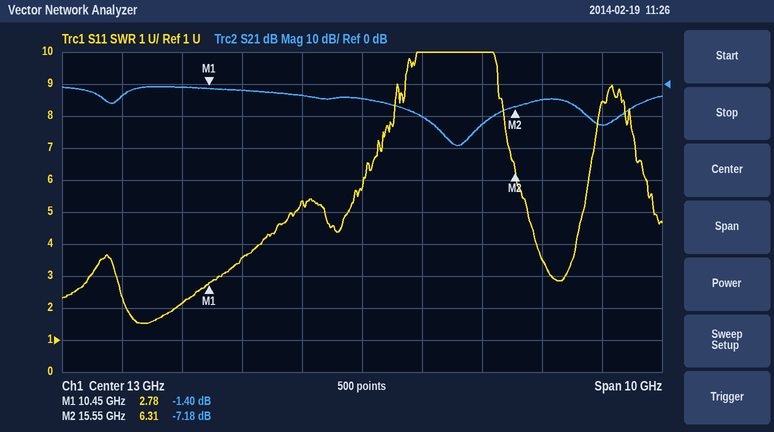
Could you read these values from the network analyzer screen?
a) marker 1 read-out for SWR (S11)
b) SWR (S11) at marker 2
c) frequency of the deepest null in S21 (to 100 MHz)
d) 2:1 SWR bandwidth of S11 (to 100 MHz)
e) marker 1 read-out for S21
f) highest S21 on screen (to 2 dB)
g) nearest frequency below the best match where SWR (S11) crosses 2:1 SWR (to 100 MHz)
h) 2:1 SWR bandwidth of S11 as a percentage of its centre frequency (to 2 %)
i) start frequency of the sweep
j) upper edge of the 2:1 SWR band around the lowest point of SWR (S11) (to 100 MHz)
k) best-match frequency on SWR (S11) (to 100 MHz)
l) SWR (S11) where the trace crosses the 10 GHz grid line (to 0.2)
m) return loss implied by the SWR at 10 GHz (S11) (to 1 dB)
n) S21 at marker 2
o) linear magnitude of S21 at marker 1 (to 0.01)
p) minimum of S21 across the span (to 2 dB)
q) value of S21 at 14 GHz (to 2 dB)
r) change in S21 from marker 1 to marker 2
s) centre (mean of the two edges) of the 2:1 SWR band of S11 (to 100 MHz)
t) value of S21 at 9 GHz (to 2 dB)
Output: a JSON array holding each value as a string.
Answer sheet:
["2.78", "6.31", "14.6 GHz", "800 MHz", "-1.40 dB", "0 dB", "9.1 GHz", "8 %", "8 GHz", "9.9 GHz", "9.3 GHz", "2.2", "9 dB", "-7.18 dB", "0.85", "-20 dB", "-10 dB", "-5.78 dB", "9.5 GHz", "-4 dB"]
